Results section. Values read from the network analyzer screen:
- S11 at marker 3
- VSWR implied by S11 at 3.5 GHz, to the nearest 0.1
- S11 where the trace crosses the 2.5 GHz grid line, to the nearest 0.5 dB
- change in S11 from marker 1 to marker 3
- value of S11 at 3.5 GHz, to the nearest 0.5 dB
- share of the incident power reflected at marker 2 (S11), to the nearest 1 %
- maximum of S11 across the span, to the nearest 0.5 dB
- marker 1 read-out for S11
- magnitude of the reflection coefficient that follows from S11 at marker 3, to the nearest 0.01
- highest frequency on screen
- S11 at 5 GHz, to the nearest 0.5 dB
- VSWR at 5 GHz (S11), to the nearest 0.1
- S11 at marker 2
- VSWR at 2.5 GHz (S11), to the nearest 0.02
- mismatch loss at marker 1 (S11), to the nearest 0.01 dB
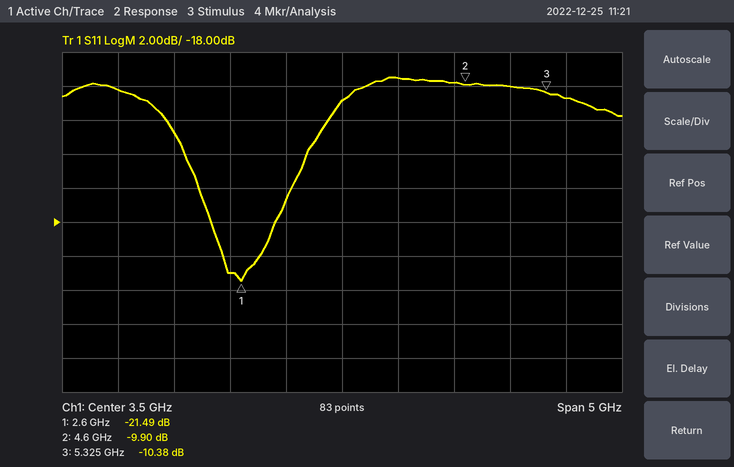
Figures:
-10.38 dB
1.8
-21.0 dB
11.11 dB
-11.0 dB
10 %
-9.5 dB
-21.49 dB
0.30
6 GHz
-10.0 dB
1.9
-9.90 dB
1.20
0.03 dB
